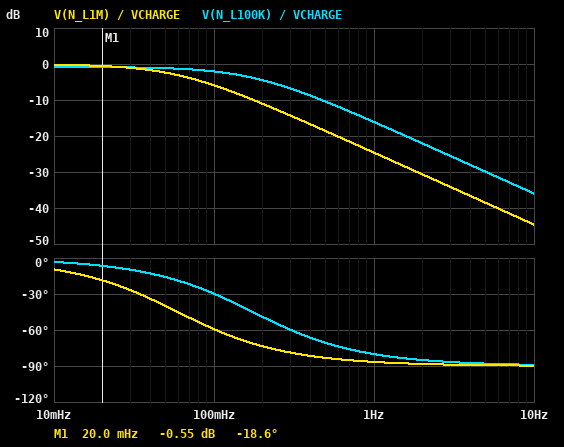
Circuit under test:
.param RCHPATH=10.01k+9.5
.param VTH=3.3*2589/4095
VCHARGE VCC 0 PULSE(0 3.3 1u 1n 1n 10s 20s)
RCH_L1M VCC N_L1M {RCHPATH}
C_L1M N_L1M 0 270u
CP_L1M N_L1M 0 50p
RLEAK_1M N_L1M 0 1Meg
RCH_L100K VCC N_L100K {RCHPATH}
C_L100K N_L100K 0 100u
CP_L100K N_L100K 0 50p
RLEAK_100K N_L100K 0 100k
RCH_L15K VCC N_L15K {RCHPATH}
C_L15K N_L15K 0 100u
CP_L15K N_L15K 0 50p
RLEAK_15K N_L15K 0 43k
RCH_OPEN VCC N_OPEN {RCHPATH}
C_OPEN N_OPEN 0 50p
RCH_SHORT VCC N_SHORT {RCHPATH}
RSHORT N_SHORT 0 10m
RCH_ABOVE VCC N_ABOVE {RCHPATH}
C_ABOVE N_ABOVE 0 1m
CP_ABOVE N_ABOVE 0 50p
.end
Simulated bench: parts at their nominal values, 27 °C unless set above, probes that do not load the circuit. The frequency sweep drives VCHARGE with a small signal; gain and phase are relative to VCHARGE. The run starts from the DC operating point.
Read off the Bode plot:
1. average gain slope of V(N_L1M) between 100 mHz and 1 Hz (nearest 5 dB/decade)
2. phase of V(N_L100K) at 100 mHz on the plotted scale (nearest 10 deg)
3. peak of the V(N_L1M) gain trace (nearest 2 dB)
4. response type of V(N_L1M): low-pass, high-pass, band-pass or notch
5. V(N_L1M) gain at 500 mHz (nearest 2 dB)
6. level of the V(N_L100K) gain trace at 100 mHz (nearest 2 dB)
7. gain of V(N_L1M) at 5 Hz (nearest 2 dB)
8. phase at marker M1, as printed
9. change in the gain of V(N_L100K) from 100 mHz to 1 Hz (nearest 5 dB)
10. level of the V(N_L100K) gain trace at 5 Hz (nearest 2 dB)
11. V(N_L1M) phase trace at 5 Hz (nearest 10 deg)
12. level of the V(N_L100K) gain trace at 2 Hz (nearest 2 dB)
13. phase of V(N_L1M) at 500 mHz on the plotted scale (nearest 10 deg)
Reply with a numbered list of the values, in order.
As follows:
1. -20 dB/decade
2. -30 deg
3. 0 dB
4. low-pass
5. -18 dB
6. -2 dB
7. -38 dB
8. -18.6 deg
9. -15 dB
10. -30 dB
11. -90 deg
12. -22 dB
13. -80 deg
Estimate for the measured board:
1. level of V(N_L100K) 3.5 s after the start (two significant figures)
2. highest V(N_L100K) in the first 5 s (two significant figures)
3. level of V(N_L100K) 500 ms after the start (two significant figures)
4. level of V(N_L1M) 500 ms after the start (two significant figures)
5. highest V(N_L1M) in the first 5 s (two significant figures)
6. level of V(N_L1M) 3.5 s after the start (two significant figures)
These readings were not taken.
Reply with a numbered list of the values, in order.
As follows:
1. 2.9 V
2. 3.0 V
3. 1.3 V
4. 560 mV
5. 2.8 V
6. 2.4 V
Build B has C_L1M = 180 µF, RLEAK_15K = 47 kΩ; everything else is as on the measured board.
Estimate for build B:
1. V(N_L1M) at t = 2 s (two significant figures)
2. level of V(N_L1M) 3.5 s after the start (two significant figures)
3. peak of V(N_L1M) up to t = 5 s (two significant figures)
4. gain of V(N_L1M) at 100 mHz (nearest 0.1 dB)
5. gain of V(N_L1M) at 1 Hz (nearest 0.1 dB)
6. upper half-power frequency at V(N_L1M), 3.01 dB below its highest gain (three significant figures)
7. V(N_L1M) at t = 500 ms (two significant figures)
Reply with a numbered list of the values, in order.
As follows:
1. 2.2 V
2. 2.8 V
3. 3.1 V
4. -3.6 dB
5. -21.1 dB
6. 89.1 mHz
7. 800 mV
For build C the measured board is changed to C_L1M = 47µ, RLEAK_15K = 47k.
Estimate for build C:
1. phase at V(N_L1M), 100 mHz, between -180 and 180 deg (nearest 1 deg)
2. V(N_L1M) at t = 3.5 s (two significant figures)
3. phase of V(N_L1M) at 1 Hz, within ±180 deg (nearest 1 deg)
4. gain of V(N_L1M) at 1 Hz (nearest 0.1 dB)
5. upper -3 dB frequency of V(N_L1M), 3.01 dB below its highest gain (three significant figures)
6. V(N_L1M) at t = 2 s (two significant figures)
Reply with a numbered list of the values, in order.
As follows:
1. -16 deg
2. 3.3 V
3. -71 deg
4. -9.9 dB
5. 341 mHz
6. 3.2 V
